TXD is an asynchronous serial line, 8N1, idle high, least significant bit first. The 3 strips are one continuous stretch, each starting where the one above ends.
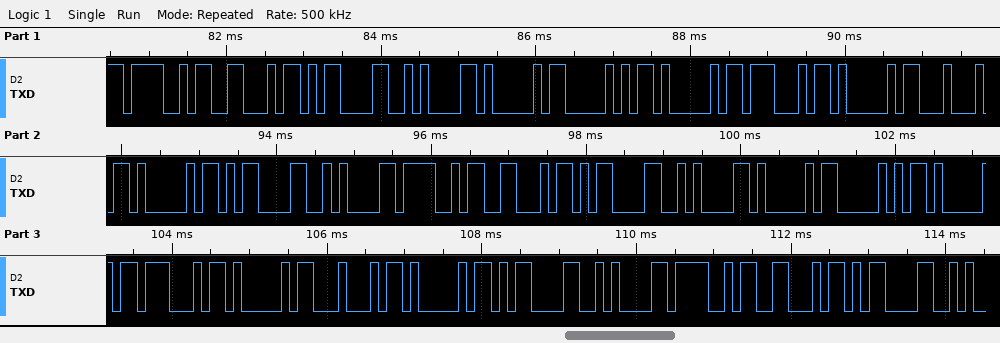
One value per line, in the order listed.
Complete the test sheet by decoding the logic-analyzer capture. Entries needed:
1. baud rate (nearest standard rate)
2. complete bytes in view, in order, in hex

9600 baud
4F 46 0D 0A 41 50 41 47 41 44 41 0D 0A 4F 46 0D 0A 41 50 41 47 41 44 41 0D 0A 4F 46 0D
